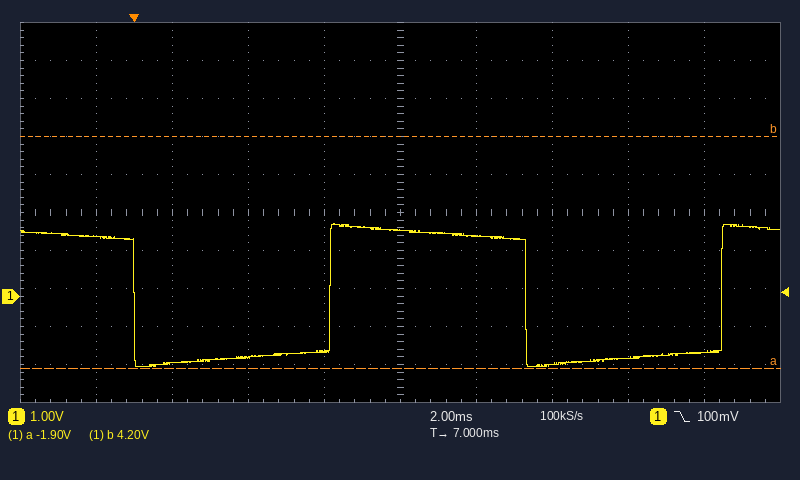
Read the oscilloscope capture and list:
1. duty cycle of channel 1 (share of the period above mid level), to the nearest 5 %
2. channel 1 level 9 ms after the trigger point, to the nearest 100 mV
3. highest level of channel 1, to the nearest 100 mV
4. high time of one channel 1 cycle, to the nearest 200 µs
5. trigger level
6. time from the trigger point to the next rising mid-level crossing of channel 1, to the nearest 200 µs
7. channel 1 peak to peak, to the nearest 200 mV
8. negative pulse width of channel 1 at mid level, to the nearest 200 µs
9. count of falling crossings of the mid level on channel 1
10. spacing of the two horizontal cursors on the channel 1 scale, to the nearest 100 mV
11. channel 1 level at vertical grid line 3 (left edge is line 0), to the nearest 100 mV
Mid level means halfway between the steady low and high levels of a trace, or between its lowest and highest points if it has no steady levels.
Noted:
50 %
1.6 V
1.9 V
5.2 ms
100 mV
5.2 ms
3.8 V
5.2 ms
2
6.1 V
-1.6 V
